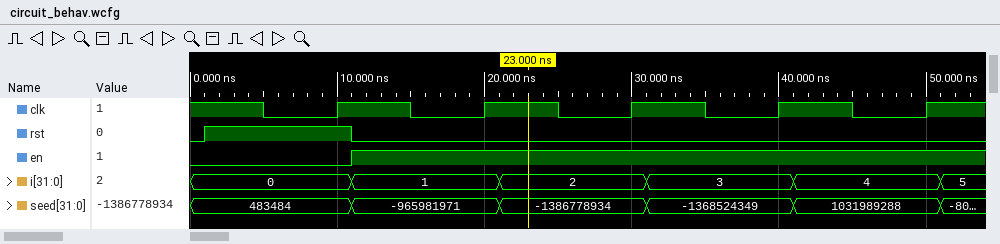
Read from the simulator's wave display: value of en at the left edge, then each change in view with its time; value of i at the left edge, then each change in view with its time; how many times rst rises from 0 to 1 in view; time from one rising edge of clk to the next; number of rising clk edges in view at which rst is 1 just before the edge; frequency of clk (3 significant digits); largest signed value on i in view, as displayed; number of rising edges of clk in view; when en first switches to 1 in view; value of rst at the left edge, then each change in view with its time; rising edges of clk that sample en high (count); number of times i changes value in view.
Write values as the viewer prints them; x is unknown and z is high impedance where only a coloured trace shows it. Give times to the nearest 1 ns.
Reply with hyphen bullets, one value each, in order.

- 0, 1 at 11 ns
- 0, 1 at 11 ns, 2 at 21 ns, 3 at 31 ns, 4 at 41 ns, 5 at 51 ns
- 1
- 10 ns
- 1
- 100 MHz
- 5
- 5
- 11 ns
- 0, 1 at 1 ns, 0 at 11 ns
- 4
- 5
